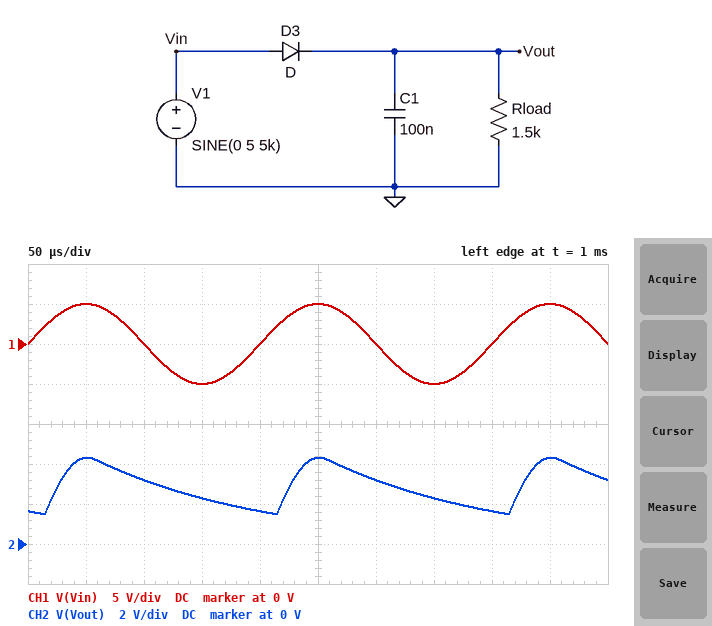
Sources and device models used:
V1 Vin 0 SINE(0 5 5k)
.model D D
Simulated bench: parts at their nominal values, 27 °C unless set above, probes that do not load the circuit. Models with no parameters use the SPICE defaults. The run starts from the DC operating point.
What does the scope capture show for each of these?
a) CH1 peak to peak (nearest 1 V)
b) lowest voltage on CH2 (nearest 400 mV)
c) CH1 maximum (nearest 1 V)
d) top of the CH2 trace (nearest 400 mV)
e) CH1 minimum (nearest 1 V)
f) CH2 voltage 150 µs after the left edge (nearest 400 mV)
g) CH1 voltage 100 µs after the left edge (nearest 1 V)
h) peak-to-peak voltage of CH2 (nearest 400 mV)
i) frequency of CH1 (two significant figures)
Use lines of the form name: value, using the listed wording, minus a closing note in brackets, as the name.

CH1 peak to peak: 10 V
lowest voltage on CH2: 1.6 V
CH1 maximum: 5 V
top of the CH2 trace: 4.4 V
CH1 minimum: -5 V
CH2 voltage 150 µs after the left edge: 2.4 V
CH1 voltage 100 µs after the left edge: 0 V
peak-to-peak voltage of CH2: 2.8 V
frequency of CH1: 5.0 kHz
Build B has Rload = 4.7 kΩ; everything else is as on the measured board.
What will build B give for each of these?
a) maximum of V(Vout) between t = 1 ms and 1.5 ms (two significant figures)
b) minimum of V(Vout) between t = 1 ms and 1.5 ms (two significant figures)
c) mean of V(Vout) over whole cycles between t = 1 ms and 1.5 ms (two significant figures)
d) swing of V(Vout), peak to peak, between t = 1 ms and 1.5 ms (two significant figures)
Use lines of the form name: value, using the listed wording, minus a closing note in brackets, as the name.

maximum of V(Vout) between t = 1 ms and 1.5 ms: 4.3 V
minimum of V(Vout) between t = 1 ms and 1.5 ms: 3.0 V
mean of V(Vout) over whole cycles between t = 1 ms and 1.5 ms: 3.7 V
swing of V(Vout), peak to peak, between t = 1 ms and 1.5 ms: 1.3 V
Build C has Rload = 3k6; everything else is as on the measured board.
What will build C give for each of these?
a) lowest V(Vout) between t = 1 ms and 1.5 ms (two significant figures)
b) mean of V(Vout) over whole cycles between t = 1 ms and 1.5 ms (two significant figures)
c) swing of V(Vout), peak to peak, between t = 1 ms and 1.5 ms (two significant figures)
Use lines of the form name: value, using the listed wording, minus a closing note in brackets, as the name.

lowest V(Vout) between t = 1 ms and 1.5 ms: 2.7 V
mean of V(Vout) over whole cycles between t = 1 ms and 1.5 ms: 3.5 V
swing of V(Vout), peak to peak, between t = 1 ms and 1.5 ms: 1.6 V
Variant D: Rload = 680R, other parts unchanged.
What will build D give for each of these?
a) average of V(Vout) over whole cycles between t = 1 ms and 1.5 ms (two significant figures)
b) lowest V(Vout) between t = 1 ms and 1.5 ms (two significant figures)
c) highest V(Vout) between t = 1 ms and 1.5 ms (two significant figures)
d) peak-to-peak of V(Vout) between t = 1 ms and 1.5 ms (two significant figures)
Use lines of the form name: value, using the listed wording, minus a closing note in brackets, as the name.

average of V(Vout) over whole cycles between t = 1 ms and 1.5 ms: 2.1 V
lowest V(Vout) between t = 1 ms and 1.5 ms: 480 mV
highest V(Vout) between t = 1 ms and 1.5 ms: 4.3 V
peak-to-peak of V(Vout) between t = 1 ms and 1.5 ms: 3.8 V
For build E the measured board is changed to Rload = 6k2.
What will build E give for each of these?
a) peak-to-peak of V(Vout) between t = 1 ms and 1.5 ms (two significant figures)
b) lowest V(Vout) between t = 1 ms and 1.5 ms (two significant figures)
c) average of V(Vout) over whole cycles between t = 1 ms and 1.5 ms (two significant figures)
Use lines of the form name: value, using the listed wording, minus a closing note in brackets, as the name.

peak-to-peak of V(Vout) between t = 1 ms and 1.5 ms: 1.1 V
lowest V(Vout) between t = 1 ms and 1.5 ms: 3.3 V
average of V(Vout) over whole cycles between t = 1 ms and 1.5 ms: 3.8 V
